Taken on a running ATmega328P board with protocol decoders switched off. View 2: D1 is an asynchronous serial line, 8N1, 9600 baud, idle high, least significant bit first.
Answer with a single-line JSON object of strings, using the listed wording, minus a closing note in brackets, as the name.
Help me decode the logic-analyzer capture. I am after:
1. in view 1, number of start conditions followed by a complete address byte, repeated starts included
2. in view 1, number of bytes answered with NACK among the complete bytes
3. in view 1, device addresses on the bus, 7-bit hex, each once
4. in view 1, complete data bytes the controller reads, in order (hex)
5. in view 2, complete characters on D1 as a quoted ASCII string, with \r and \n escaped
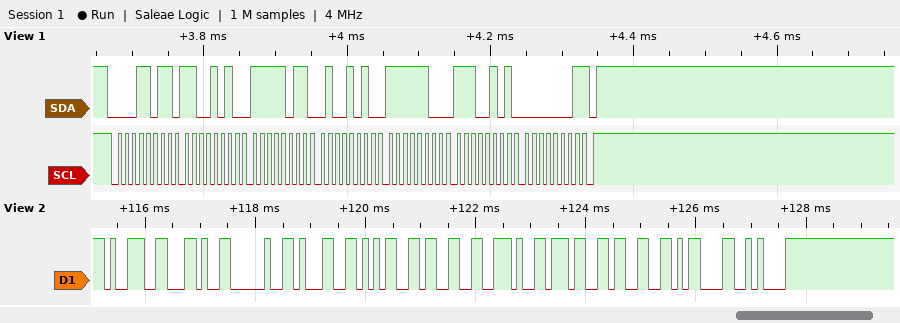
{"in view 1, number of start conditions followed by a complete address byte, repeated starts included": "1", "in view 1, number of bytes answered with NACK among the complete bytes": "1", "in view 1, device addresses on the bus, 7-bit hex, each once": "0x0D", "in view 1, complete data bytes the controller reads, in order": "CA FB 4A FC E5 01", "in view 2, complete characters on D1 as a quoted ASCII string, with \\r and \\n escaped": "\"9, 153.73\\r\\n\""}
